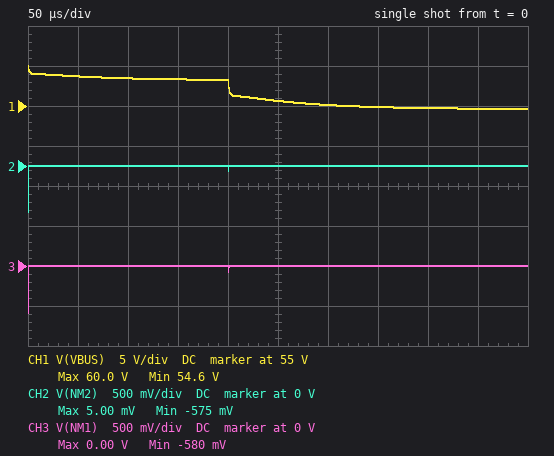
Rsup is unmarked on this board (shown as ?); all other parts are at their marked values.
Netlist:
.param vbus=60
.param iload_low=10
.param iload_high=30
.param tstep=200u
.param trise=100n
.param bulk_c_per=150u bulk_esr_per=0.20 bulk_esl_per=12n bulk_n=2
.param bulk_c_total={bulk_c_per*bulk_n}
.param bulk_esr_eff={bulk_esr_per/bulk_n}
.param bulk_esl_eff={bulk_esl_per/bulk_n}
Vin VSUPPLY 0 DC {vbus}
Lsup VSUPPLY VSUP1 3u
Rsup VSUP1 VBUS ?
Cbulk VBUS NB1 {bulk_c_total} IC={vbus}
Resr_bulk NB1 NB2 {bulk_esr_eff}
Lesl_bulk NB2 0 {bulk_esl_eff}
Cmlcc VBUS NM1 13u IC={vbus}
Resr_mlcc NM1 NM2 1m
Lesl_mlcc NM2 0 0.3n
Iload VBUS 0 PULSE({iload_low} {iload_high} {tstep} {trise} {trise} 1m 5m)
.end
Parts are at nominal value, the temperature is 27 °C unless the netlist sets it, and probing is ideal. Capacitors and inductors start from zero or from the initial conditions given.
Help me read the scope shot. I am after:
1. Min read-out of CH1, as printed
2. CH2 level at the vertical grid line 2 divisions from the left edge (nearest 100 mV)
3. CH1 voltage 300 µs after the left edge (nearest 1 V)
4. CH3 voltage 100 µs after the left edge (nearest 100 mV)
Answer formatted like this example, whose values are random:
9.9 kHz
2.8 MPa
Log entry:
54.6 V
0 V
55 V
0 V
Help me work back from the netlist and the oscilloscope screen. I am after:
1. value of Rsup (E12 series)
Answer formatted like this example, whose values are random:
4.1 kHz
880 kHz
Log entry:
0.18 Ω
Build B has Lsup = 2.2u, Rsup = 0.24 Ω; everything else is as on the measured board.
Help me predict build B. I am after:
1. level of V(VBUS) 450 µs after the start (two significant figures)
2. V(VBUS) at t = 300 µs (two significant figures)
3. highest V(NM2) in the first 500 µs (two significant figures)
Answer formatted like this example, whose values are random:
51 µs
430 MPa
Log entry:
53 V
54 V
4.0 mV
